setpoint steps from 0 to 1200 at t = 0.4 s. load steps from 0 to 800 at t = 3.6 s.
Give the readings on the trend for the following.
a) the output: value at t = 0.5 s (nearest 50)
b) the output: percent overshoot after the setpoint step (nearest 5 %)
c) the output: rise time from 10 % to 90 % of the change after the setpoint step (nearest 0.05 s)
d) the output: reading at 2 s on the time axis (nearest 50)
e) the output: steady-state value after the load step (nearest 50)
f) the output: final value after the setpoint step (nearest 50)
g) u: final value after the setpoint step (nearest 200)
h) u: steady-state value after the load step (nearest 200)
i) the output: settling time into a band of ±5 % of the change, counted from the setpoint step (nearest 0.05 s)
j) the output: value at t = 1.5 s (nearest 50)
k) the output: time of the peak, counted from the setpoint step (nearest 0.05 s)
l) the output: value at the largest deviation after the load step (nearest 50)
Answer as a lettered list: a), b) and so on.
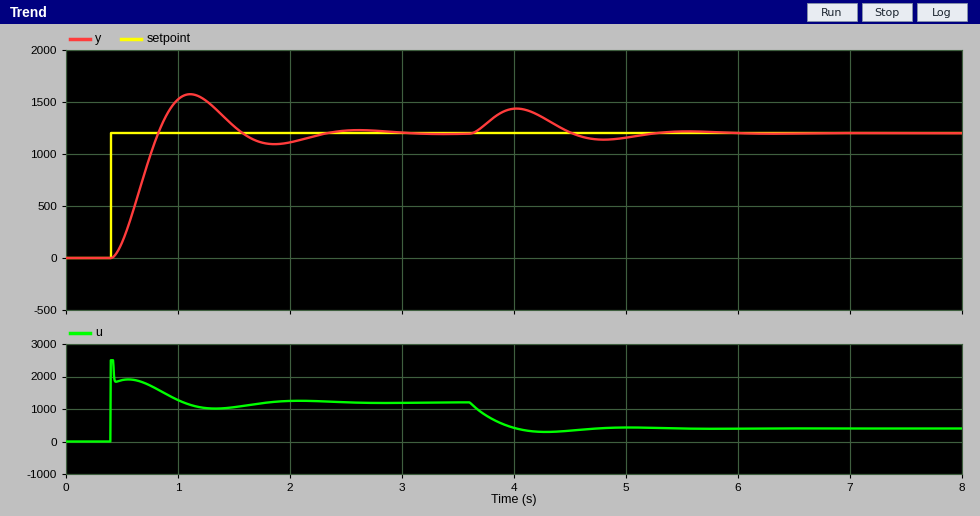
a) 150
b) 30 %
c) 0.30 s
d) 1100
e) 1200
f) 1200
g) 1200
h) 400
i) 1.70 s
j) 1250
k) 0.70 s
l) 1450
